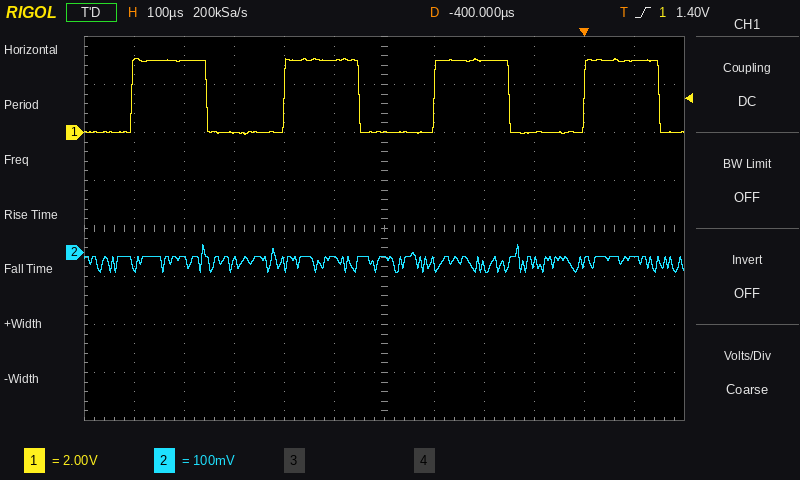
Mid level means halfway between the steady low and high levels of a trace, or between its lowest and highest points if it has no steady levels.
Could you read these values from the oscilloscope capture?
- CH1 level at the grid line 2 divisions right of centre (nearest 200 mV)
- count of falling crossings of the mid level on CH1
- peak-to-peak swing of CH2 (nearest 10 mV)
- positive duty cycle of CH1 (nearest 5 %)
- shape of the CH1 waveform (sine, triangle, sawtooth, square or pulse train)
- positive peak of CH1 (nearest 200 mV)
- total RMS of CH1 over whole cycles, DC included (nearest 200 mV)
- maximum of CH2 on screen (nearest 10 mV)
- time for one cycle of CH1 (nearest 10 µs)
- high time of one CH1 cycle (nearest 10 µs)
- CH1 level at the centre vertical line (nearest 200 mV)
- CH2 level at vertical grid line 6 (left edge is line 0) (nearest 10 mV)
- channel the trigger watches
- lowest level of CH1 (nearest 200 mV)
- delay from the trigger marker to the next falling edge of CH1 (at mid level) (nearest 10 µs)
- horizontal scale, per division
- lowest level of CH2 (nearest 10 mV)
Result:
3.0 V
4
60 mV
50 %
square
3.0 V
2.2 V
20 mV
300 µs
150 µs
0.0 V
-10 mV
CH1
0.0 V
150 µs
100 µs
-40 mV
